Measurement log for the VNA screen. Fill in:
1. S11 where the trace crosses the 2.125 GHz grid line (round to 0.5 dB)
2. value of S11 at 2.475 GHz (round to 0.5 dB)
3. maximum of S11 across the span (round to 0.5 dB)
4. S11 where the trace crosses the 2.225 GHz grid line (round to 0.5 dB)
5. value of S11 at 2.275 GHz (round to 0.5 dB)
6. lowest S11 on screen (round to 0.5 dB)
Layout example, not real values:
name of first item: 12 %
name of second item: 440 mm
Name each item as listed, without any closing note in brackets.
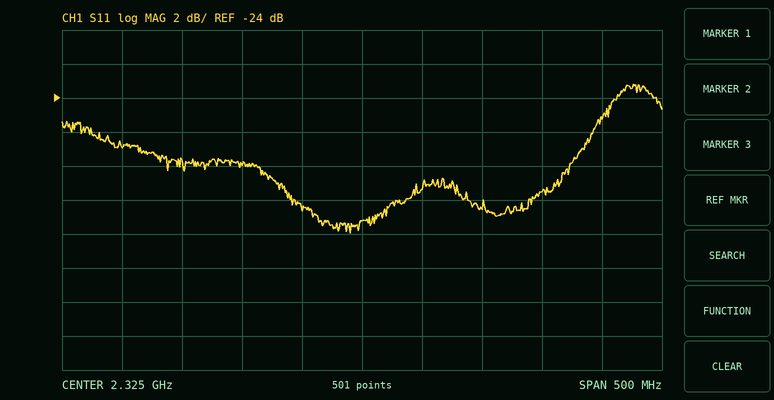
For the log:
S11 where the trace crosses the 2.125 GHz grid line: -27.0 dB
value of S11 at 2.475 GHz: -29.5 dB
maximum of S11 across the span: -23.0 dB
S11 where the trace crosses the 2.225 GHz grid line: -28.0 dB
value of S11 at 2.275 GHz: -30.5 dB
lowest S11 on screen: -32.0 dB
